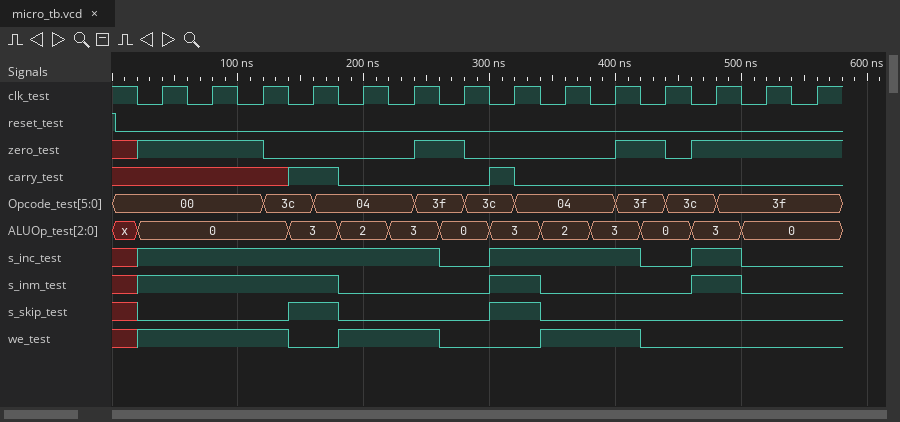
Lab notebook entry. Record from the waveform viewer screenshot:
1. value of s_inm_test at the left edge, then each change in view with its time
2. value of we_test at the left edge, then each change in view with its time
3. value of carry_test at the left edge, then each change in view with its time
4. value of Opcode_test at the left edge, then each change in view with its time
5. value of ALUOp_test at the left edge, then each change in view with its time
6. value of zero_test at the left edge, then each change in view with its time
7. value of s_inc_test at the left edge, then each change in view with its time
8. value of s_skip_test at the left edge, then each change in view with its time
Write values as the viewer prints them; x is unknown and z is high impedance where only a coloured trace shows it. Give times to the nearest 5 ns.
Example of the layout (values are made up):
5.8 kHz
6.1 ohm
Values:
x, 1 at 20 ns, 0 at 180 ns, 1 at 300 ns, 0 at 340 ns, 1 at 460 ns, 0 at 500 ns
x, 1 at 20 ns, 0 at 140 ns, 1 at 180 ns, 0 at 260 ns, 1 at 340 ns, 0 at 420 ns
x, 1 at 140 ns, 0 at 180 ns, 1 at 300 ns, 0 at 320 ns
00, 3c at 120 ns, 04 at 160 ns, 3f at 240 ns, 3c at 280 ns, 04 at 320 ns, 3f at 400 ns, 3c at 440 ns, 3f at 480 ns
x, 0 at 20 ns, 3 at 140 ns, 2 at 180 ns, 3 at 220 ns, 0 at 260 ns, 3 at 300 ns, 2 at 340 ns, 3 at 380 ns, 0 at 420 ns, 3 at 460 ns, 0 at 500 ns
x, 1 at 20 ns, 0 at 120 ns, 1 at 240 ns, 0 at 280 ns, 1 at 400 ns, 0 at 440 ns, 1 at 460 ns
x, 1 at 20 ns, 0 at 260 ns, 1 at 300 ns, 0 at 420 ns, 1 at 460 ns, 0 at 500 ns
x, 0 at 20 ns, 1 at 140 ns, 0 at 180 ns, 1 at 300 ns, 0 at 340 ns
